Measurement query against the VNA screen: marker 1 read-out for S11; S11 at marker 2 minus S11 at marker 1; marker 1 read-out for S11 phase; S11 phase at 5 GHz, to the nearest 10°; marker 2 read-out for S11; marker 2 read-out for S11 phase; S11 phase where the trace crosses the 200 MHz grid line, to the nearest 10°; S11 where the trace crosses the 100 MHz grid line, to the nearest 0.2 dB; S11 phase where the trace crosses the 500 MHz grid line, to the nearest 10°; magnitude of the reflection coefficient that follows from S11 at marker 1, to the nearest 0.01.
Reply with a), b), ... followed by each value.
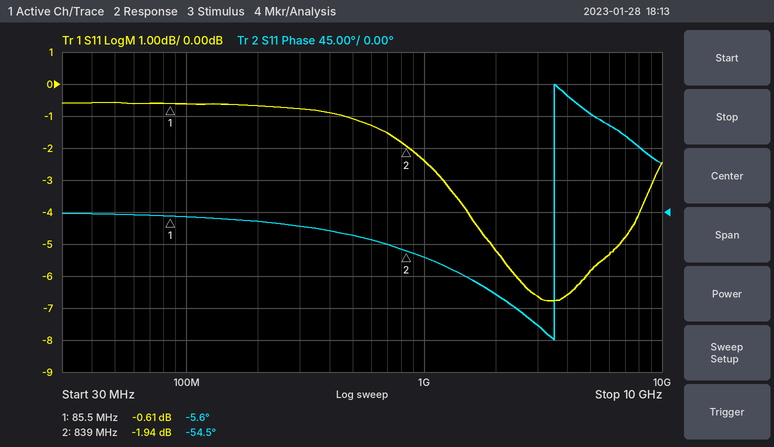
a) -0.61 dB
b) -1.33 dB
c) -5.6°
d) 140°
e) -1.94 dB
f) -54.5°
g) -10°
h) -0.6 dB
i) -30°
j) 0.93
